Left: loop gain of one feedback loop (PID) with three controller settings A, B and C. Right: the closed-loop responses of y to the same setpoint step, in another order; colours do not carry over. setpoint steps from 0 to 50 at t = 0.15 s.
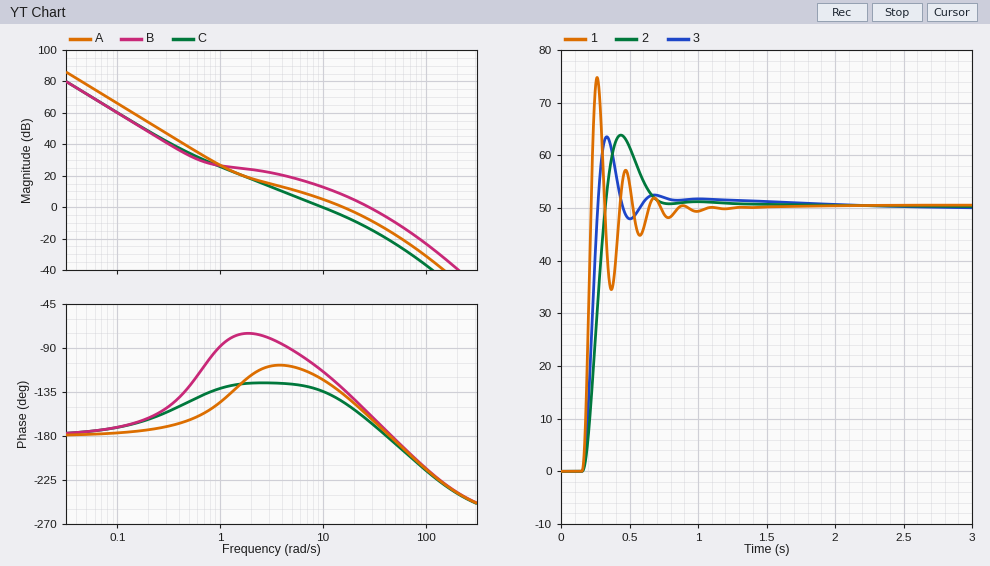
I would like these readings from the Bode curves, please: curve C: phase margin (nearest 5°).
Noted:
45°
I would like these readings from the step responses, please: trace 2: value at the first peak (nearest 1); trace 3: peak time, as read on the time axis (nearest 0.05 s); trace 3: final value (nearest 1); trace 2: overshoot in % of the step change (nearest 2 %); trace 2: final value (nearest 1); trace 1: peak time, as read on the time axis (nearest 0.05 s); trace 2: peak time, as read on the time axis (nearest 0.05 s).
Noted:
64
0.35 s
50
28 %
50
0.25 s
0.45 s
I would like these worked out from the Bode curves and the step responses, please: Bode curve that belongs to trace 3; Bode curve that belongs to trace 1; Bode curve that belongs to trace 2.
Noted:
A
B
C
